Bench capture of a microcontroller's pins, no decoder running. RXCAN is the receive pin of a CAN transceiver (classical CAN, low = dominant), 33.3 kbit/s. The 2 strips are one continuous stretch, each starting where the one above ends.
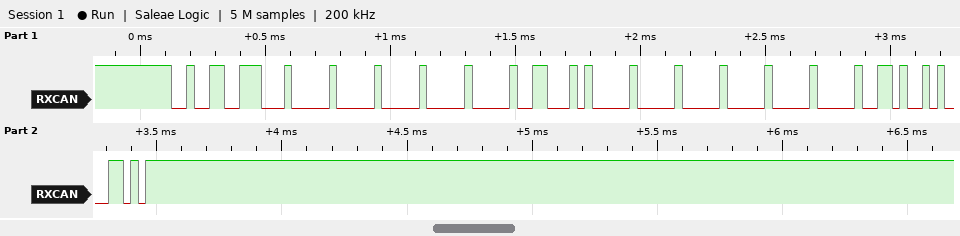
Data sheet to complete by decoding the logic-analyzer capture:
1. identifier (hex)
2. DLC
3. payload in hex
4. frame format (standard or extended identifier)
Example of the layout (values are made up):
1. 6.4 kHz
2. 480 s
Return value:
1. 0x267
2. 8
3. 00 00 00 C5 00 00 00 00
4. standard
